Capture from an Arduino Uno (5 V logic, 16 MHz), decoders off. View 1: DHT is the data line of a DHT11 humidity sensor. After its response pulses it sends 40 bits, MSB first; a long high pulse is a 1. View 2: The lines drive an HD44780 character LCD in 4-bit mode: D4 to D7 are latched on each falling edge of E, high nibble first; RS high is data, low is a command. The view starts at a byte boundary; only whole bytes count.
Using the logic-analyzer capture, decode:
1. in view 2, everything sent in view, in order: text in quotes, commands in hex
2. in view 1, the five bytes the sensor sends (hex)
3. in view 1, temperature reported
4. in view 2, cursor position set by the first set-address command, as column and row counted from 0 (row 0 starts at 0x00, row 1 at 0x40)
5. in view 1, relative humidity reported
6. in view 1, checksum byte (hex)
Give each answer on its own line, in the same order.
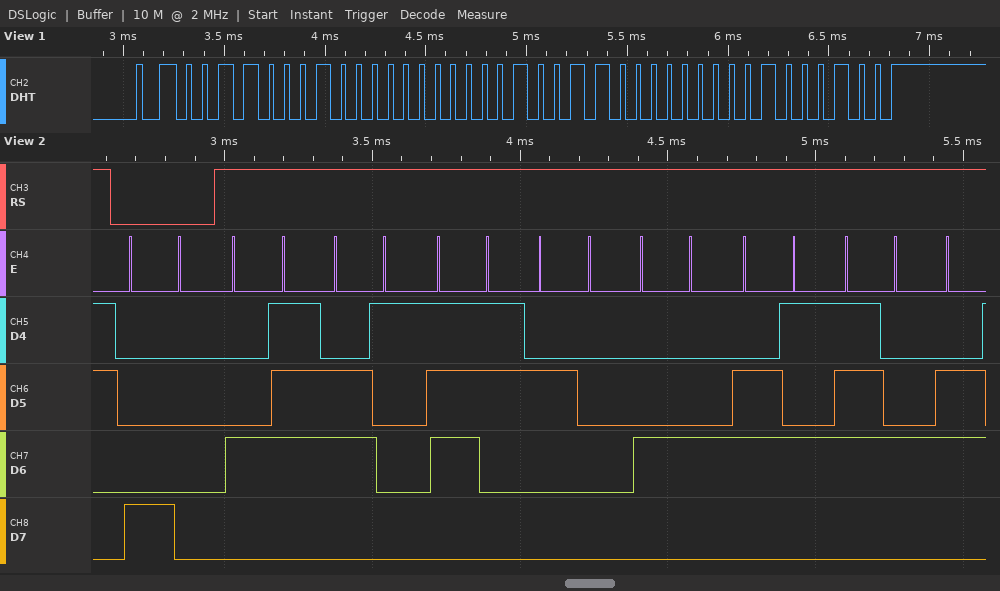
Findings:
0x80 "Gas Det"
31 00 13 00 44
19.0 °C
column 0, row 0
49 %
0x44
